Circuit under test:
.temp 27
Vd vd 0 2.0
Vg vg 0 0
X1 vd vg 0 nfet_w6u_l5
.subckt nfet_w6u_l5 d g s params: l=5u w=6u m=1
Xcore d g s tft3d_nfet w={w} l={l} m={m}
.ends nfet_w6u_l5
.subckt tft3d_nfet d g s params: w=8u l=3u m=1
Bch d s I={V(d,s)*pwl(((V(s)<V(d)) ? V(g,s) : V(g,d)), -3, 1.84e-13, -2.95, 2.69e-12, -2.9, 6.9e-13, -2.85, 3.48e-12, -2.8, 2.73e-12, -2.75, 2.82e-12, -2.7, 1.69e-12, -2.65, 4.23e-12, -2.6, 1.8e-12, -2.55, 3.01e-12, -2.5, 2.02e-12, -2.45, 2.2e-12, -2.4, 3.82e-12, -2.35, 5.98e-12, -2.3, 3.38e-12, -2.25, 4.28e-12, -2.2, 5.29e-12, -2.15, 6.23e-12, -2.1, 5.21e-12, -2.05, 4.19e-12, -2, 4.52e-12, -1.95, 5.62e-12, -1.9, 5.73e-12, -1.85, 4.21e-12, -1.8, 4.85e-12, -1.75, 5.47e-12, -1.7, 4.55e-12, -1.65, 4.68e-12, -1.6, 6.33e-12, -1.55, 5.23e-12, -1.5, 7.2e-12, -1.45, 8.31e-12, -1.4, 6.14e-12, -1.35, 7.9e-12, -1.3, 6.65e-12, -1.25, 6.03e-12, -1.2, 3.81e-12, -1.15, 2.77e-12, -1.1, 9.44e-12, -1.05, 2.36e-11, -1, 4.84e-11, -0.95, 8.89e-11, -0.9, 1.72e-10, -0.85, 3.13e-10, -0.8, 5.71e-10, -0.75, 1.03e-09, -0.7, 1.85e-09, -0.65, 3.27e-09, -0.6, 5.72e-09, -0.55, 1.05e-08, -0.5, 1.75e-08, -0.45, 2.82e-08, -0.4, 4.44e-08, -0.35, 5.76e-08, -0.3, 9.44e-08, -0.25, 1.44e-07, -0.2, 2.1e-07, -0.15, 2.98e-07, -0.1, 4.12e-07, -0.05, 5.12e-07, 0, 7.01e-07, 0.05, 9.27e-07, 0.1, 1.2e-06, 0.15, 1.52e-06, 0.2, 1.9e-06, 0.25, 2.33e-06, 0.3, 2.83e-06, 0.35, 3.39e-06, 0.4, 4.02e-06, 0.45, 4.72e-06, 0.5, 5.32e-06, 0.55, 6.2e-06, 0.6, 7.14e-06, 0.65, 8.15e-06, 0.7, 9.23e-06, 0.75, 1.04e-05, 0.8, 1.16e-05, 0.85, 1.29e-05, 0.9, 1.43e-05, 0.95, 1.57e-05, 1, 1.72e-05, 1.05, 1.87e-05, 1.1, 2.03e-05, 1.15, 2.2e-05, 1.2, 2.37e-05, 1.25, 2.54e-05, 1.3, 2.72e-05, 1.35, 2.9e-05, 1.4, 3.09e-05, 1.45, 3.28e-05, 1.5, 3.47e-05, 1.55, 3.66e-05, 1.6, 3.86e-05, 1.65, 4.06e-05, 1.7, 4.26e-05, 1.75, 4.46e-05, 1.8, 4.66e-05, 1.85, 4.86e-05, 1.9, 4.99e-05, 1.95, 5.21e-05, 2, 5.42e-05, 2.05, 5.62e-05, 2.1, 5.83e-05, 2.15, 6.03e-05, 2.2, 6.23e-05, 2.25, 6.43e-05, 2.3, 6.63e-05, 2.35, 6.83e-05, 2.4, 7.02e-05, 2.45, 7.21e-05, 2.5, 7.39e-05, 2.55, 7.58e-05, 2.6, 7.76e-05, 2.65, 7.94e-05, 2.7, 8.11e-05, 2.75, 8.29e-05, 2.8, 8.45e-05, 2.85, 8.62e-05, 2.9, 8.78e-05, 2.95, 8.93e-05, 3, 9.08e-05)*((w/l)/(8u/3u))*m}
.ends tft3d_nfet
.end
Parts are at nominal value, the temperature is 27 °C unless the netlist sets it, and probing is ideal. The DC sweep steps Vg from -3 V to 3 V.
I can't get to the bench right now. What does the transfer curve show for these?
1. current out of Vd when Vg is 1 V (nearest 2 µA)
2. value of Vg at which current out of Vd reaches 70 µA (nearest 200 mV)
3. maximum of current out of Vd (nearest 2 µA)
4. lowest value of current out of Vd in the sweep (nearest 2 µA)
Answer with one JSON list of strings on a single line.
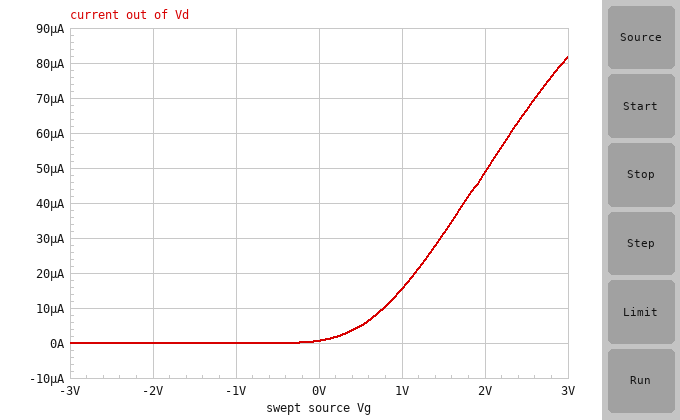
["16 µA", "2.6 V", "82 µA", "0 A"]
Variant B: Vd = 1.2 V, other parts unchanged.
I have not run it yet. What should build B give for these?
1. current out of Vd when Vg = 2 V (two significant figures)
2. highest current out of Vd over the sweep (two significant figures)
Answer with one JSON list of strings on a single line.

["29 µA", "49 µA"]
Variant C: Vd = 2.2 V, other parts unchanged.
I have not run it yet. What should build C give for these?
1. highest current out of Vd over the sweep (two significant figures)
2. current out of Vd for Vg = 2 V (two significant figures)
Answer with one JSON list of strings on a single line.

["90 µA", "54 µA"]
